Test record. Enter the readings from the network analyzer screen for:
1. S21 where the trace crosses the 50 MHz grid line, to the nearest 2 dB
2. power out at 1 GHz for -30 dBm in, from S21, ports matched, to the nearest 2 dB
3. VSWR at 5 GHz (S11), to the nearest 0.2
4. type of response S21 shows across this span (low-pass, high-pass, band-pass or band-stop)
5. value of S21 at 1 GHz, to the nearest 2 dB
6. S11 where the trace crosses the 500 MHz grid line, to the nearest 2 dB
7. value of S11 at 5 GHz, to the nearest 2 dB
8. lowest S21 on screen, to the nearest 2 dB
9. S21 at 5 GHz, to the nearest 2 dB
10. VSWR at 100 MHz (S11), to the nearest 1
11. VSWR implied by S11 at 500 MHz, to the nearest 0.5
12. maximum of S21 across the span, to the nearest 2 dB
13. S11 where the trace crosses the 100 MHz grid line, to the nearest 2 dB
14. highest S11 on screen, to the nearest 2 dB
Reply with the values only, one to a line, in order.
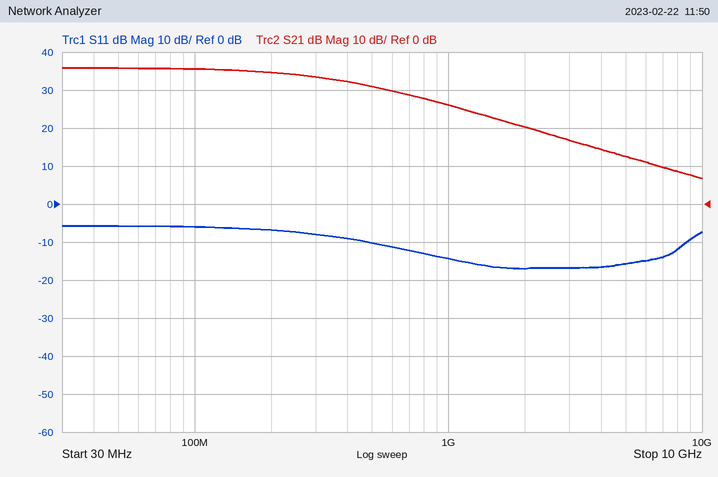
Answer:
36 dB
-4 dBm
1.4
low-pass
26 dB
-10 dB
-16 dB
6 dB
12 dB
3
2.0
36 dB
-6 dB
-6 dB
